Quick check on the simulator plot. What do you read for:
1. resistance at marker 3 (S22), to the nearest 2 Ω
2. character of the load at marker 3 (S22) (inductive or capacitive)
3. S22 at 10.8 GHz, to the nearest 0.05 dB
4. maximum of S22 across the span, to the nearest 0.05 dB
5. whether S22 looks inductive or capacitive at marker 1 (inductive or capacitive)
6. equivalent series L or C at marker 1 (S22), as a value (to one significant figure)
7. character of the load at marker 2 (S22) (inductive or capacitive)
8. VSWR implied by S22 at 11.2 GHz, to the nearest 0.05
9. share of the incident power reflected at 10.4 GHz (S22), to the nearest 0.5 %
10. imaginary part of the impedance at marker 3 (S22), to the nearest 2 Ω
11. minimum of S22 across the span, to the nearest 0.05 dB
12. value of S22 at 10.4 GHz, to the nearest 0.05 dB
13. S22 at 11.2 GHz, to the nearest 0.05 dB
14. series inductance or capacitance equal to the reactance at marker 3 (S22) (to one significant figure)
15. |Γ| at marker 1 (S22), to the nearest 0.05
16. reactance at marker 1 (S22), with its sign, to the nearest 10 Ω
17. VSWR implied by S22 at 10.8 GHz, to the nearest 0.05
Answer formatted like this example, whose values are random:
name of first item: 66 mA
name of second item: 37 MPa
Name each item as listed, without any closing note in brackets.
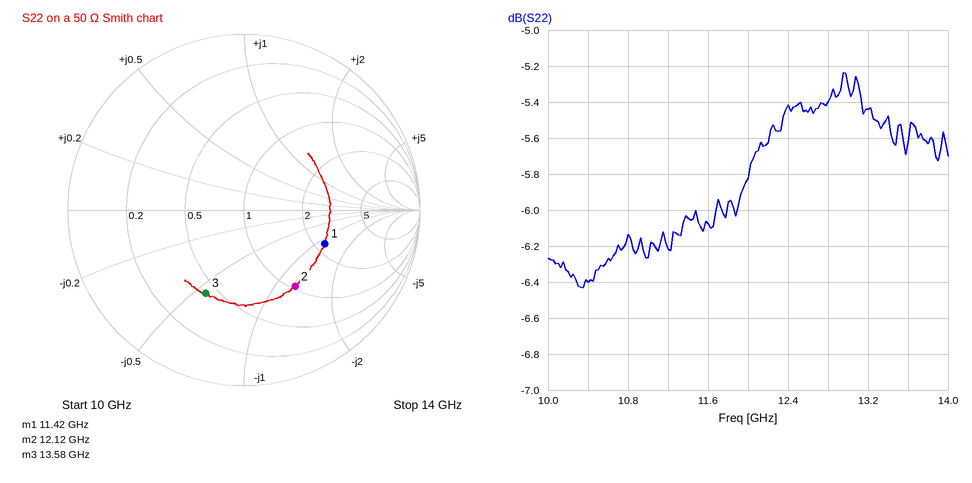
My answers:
resistance at marker 3 (S22), to the nearest 2 Ω: 22 Ω
character of the load at marker 3 (S22): capacitive
S22 at 10.8 GHz, to the nearest 0.05 dB: -6.15 dB
maximum of S22 across the span, to the nearest 0.05 dB: -5.25 dB
whether S22 looks inductive or capacitive at marker 1: capacitive
equivalent series L or C at marker 1 (S22), as a value: 200 fF
character of the load at marker 2 (S22): capacitive
VSWR implied by S22 at 11.2 GHz, to the nearest 0.05: 2.90
share of the incident power reflected at 10.4 GHz (S22), to the nearest 0.5 %: 23.0 %
imaginary part of the impedance at marker 3 (S22), to the nearest 2 Ω: -28 Ω
minimum of S22 across the span, to the nearest 0.05 dB: -6.45 dB
value of S22 at 10.4 GHz, to the nearest 0.05 dB: -6.40 dB
S22 at 11.2 GHz, to the nearest 0.05 dB: -6.20 dB
series inductance or capacitance equal to the reactance at marker 3 (S22): 400 fF
|Γ| at marker 1 (S22), to the nearest 0.05: 0.50
reactance at marker 1 (S22), with its sign, to the nearest 10 Ω: -60 Ω
VSWR implied by S22 at 10.8 GHz, to the nearest 0.05: 2.95
